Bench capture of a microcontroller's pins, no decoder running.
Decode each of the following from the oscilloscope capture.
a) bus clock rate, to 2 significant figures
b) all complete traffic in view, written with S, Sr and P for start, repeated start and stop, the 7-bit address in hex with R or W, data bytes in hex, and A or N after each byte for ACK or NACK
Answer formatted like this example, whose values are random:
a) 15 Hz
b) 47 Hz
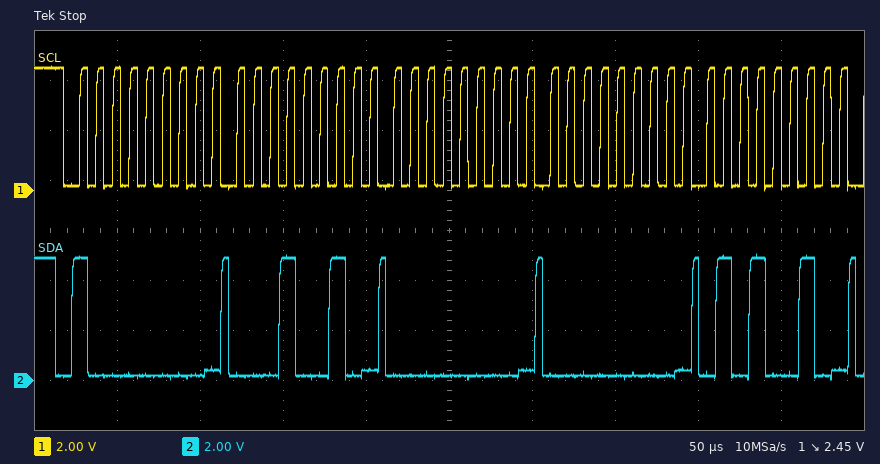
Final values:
a) 100 kHz
b) S 40W A 12 A 00 A 00 A 52 A
